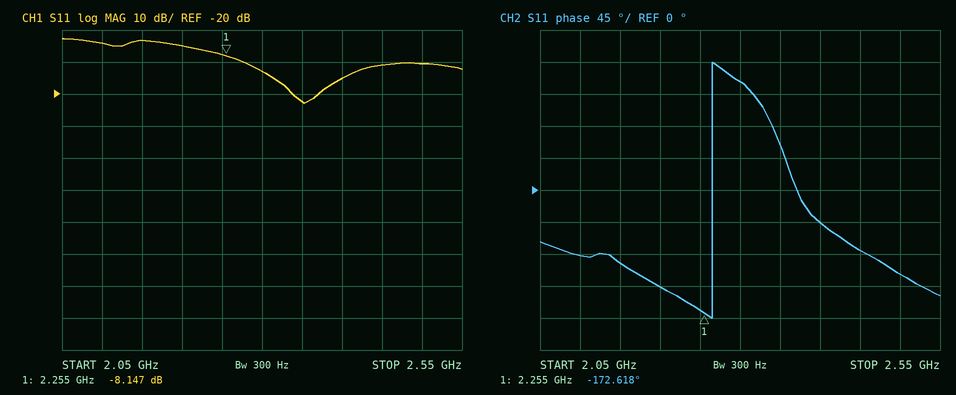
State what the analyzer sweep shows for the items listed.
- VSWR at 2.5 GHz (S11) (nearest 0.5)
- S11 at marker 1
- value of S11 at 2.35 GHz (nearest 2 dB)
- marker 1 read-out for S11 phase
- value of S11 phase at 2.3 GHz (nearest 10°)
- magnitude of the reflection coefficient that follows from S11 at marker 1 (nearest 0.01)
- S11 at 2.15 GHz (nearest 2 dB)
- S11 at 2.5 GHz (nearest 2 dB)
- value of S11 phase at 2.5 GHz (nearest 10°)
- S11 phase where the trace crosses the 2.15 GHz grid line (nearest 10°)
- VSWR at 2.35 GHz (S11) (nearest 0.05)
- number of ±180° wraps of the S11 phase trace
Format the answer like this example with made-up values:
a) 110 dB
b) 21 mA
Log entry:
a) 2.0
b) -8.147 dB
c) -22 dB
d) -172.618°
e) 150°
f) 0.39
g) -4 dB
h) -10 dB
i) -120°
j) -100°
k) 1.15
l) 1
